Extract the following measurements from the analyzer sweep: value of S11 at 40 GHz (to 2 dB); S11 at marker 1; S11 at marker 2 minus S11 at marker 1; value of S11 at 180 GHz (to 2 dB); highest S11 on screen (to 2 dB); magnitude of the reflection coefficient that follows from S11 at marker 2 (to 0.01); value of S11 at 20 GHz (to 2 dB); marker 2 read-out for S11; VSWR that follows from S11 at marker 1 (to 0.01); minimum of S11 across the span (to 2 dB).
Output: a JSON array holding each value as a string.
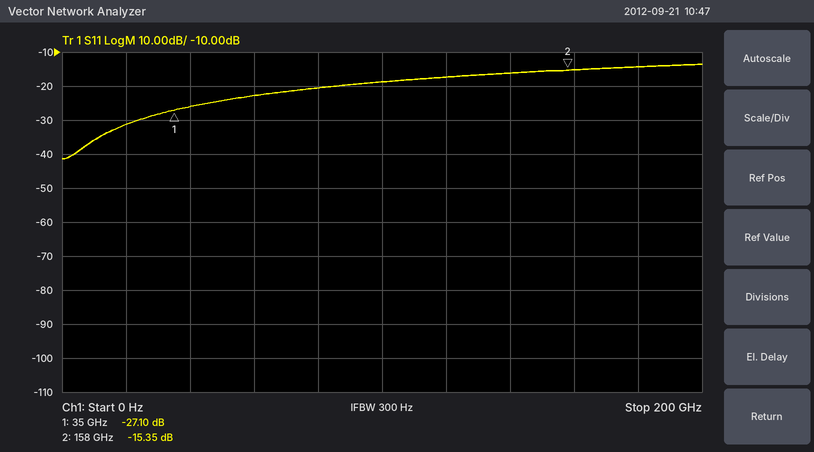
["-26 dB", "-27.10 dB", "11.75 dB", "-14 dB", "-14 dB", "0.17", "-32 dB", "-15.35 dB", "1.09", "-42 dB"]
